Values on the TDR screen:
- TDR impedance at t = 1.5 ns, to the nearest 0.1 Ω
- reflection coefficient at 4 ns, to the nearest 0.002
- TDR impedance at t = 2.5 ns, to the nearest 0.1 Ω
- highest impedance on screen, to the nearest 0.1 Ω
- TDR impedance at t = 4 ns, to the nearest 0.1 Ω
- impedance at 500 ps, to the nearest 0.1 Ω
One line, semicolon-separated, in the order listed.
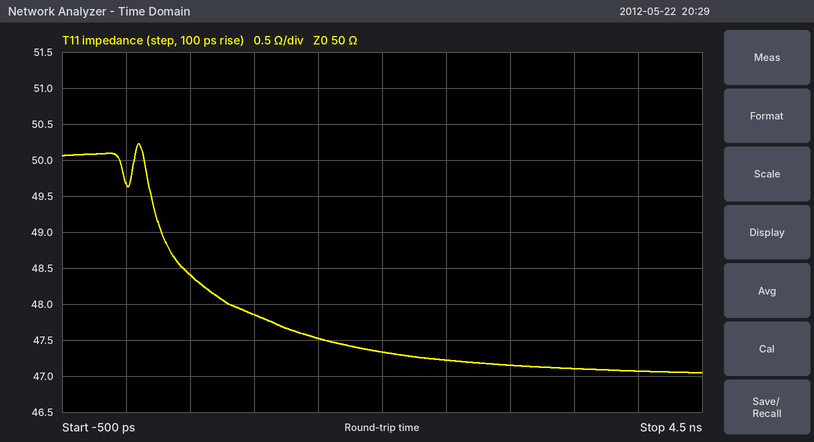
47.5 Ω; -0.030; 47.2 Ω; 50.2 Ω; 47.1 Ω; 48.4 Ω
